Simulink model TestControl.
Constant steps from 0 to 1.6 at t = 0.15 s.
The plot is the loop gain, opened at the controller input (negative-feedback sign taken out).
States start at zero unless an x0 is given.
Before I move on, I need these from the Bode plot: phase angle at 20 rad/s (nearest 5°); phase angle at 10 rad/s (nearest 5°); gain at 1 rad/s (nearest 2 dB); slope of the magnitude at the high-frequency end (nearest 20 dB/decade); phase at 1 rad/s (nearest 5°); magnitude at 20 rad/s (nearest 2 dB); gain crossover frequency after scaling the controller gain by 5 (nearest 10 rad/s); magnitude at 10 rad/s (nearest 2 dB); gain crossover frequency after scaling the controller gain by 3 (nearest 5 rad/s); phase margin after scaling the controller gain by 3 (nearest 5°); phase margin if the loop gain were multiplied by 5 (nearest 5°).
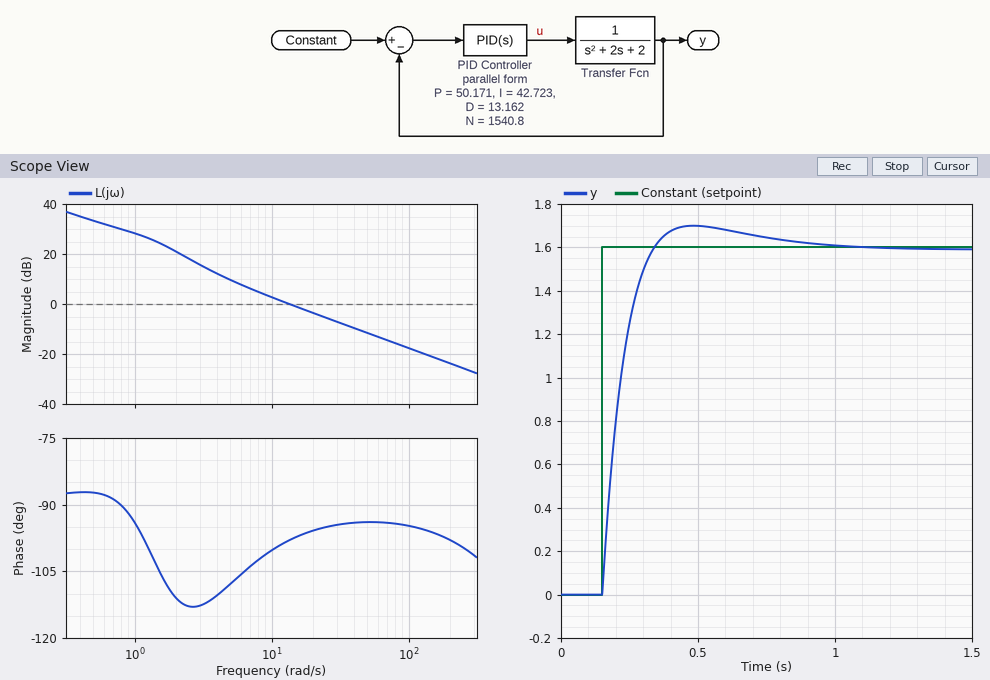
-95°
-100°
28 dB
-20 dB/decade
-95°
-4 dB
70 rad/s
2 dB
40 rad/s
85°
85°
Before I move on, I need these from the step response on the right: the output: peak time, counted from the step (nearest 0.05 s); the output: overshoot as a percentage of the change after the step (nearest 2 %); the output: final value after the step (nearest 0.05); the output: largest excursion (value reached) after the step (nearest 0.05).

0.35 s
6 %
1.60
1.70
